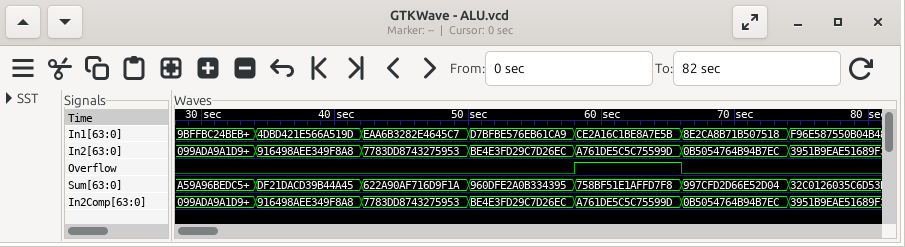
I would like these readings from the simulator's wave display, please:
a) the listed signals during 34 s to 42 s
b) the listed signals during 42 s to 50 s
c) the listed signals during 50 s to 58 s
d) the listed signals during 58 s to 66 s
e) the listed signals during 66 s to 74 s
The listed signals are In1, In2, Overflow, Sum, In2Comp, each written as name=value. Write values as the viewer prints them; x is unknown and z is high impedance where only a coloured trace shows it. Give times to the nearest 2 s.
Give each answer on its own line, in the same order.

In1=4DBD421E566A519D, In2=916498AEE349F8A8, Overflow=0, Sum=DF21DACD39B44A45, In2Comp=916498AEE349F8A8
In1=EAA6B3282E4645C7, In2=7783DD8743275953, Overflow=0, Sum=622A90AF716D9F1A, In2Comp=7783DD8743275953
In1=D7BFBE576EB61CA9, In2=BE4E3FD29C7D26EC, Overflow=0, Sum=960DFE2A0B334395, In2Comp=BE4E3FD29C7D26EC
In1=CE2A16C1BE8A7E5B, In2=A761DE5C5C75599D, Overflow=1, Sum=758BF51E1AFFD7F8, In2Comp=A761DE5C5C75599D
In1=8E2CA8B71B507518, In2=0B5054764B94B7EC, Overflow=0, Sum=997CFD2D66E52D04, In2Comp=0B5054764B94B7EC
